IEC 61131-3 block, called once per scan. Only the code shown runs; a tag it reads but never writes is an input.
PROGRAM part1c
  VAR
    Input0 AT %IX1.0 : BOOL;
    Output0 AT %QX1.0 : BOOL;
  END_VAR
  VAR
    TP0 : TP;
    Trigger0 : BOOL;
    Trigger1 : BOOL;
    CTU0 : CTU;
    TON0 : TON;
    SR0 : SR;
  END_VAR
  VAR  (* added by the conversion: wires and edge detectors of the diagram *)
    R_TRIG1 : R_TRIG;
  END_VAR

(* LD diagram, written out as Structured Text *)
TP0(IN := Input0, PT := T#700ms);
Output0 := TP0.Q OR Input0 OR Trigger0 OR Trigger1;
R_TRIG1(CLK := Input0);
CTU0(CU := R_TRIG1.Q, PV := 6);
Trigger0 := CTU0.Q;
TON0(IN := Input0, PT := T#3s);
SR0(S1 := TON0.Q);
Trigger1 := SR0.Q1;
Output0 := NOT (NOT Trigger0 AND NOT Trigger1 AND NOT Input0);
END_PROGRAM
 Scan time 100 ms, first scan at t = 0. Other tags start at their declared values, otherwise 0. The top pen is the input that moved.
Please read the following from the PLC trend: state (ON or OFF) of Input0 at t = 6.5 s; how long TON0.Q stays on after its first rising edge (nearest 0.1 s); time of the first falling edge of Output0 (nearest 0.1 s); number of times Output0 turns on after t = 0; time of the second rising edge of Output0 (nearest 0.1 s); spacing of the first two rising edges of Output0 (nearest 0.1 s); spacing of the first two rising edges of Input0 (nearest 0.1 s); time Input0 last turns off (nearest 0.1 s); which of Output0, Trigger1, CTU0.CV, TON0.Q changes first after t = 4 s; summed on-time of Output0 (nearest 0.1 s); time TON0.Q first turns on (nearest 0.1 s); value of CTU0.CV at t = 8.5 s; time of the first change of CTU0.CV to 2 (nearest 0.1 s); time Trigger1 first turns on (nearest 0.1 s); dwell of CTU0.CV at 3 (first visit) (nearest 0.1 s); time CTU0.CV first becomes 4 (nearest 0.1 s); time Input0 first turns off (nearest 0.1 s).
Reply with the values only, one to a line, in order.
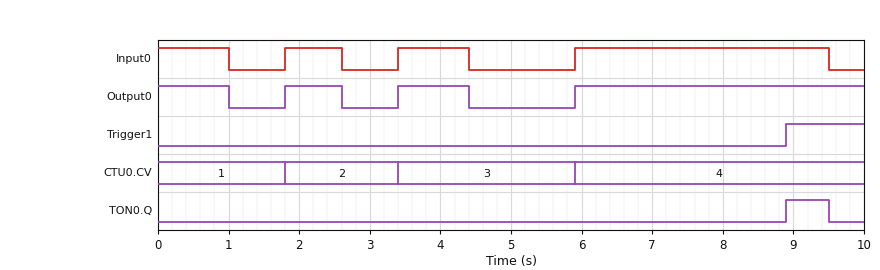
ON
0.6 s
1.0 s
3
3.4 s
1.6 s
1.6 s
9.5 s
Output0
6.9 s
8.9 s
4
1.8 s
8.9 s
2.5 s
5.9 s
1.0 s
